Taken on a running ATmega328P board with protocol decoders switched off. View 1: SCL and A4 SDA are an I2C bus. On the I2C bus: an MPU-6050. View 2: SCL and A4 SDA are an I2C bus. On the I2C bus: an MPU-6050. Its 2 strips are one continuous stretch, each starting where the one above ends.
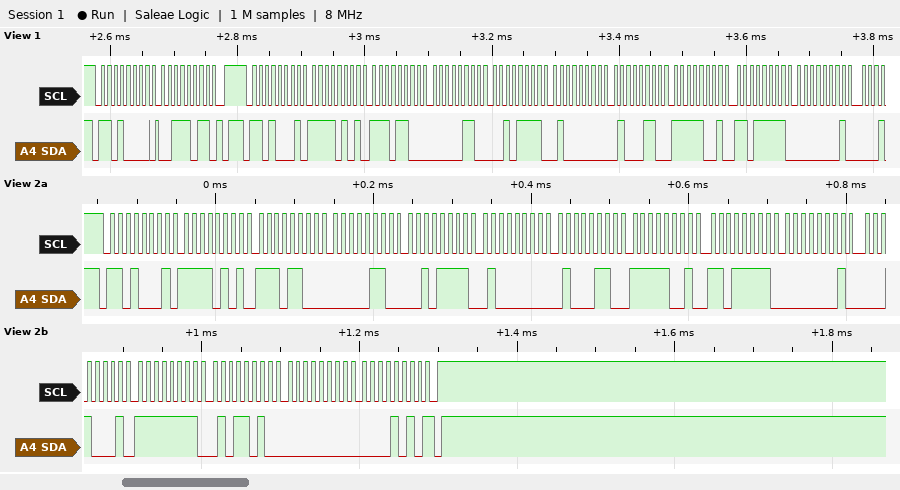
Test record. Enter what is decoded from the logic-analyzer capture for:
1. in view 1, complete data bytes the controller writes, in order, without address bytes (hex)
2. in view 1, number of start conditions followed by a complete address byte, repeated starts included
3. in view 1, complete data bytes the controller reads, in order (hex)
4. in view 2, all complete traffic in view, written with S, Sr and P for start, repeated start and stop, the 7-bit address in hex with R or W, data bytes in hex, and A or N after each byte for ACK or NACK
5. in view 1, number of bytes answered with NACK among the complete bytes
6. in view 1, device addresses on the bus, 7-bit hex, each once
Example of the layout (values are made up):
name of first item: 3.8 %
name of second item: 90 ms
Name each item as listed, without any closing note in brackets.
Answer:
in view 1, complete data bytes the controller writes, in order, without address bytes: 3B
in view 1, number of start conditions followed by a complete address byte, repeated starts included: 2
in view 1, complete data bytes the controller reads, in order: F5 EC 06 2F 40 46 F9 DF 01
in view 2, all complete traffic in view, written with S, Sr and P for start, repeated start and stop, the 7-bit address in hex with R or W, data bytes in hex, and A or N after each byte for ACK or NACK: S 68R A F5 A EC A 06 A 2F A 40 A 46 A F9 A DF A 01 A 11 A FF A 5A A 00 A 0A N P
in view 1, number of bytes answered with NACK among the complete bytes: 0
in view 1, device addresses on the bus, 7-bit hex, each once: 0x68
